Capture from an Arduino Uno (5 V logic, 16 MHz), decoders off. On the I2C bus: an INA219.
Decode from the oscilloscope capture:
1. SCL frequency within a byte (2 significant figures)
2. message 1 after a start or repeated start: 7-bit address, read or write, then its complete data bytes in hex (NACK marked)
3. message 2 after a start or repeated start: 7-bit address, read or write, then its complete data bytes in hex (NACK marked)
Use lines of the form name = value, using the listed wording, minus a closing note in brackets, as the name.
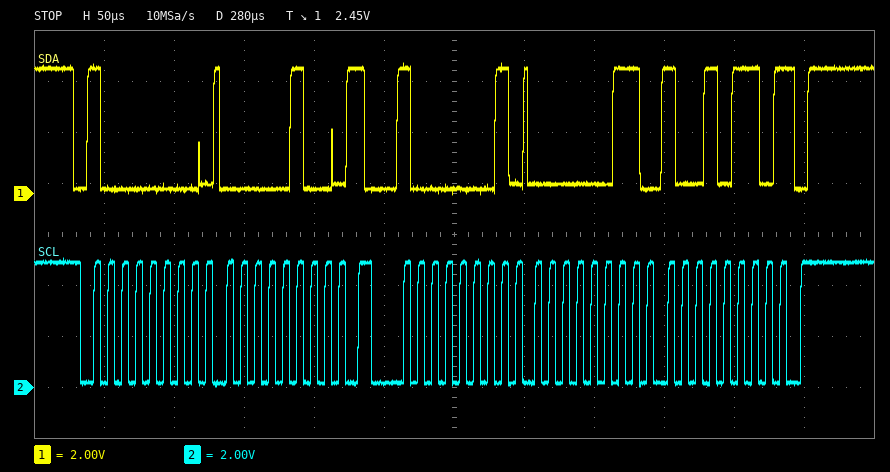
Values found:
SCL frequency within a byte = 100 kHz
message 1 after a start or repeated start: 7-bit address, read or write, then its complete data bytes in hex = 0x40 write: 04
message 2 after a start or repeated start: 7-bit address, read or write, then its complete data bytes in hex = 0x40 read: 03 96 NACK
